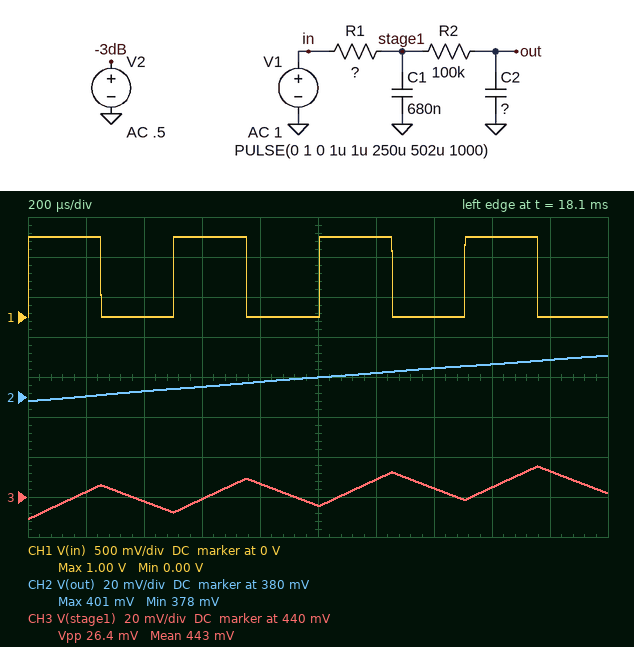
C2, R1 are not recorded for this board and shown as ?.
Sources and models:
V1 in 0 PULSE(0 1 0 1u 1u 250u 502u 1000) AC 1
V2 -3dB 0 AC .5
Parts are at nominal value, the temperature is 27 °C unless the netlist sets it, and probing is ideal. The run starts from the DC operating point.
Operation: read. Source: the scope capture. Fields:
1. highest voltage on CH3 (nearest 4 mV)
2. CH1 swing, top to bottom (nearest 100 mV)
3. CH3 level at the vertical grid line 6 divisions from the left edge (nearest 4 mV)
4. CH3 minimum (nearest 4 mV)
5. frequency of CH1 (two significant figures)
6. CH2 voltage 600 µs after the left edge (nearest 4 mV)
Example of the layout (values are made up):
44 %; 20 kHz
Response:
456 mV; 1.0 V; 448 mV; 428 mV; 2.0 kHz; 384 mV
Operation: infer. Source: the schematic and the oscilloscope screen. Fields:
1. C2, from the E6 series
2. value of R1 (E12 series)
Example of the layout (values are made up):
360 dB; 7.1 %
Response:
47 nF; 12 kΩ
